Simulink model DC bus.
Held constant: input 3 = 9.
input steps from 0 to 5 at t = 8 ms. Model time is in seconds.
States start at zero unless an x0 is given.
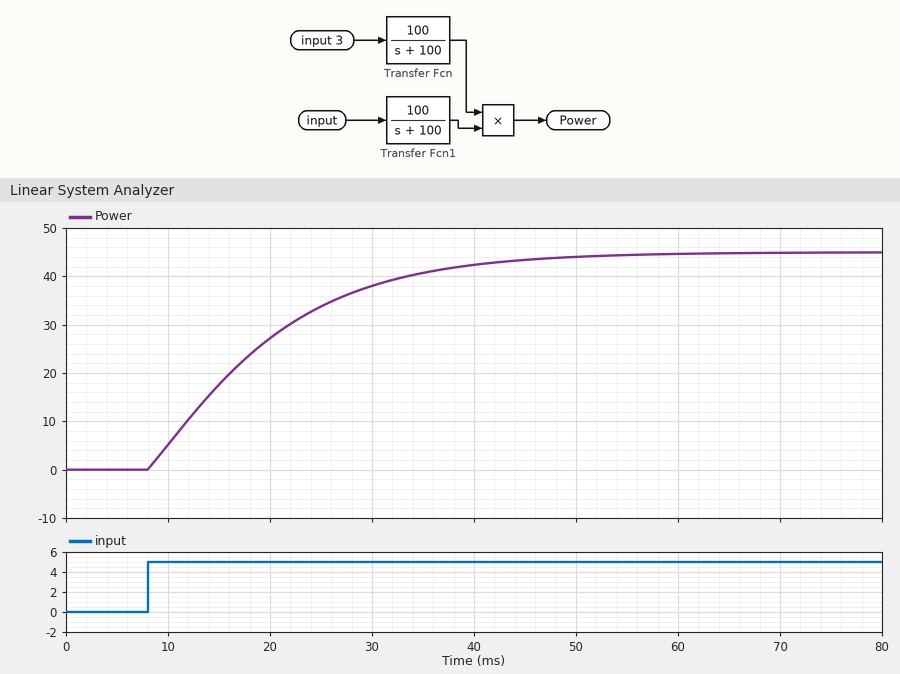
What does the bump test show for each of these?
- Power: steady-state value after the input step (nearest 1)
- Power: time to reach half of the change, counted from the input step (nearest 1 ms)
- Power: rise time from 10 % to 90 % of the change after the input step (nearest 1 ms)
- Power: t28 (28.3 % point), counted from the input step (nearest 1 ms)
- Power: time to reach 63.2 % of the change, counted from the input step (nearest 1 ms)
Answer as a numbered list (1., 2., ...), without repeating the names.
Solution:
1. 45
2. 9 ms
3. 25 ms
4. 5 ms
5. 13 ms
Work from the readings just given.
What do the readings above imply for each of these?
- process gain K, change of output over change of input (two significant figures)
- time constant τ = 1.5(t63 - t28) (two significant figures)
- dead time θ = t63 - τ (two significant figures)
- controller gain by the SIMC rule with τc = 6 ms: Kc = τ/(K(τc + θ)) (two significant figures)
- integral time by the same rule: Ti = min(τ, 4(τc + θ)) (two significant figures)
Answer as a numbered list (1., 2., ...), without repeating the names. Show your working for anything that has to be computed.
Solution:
1. (45 - 0) / 5 = 9.0
2. 1.5 × (13 - 5) = 12 ms
3. 13 - 12 = 1.0 ms
4. 12 / (9 × (6 + 1)) = 0.19
5. min(12, 4 × (6 + 1)) = 12 ms
